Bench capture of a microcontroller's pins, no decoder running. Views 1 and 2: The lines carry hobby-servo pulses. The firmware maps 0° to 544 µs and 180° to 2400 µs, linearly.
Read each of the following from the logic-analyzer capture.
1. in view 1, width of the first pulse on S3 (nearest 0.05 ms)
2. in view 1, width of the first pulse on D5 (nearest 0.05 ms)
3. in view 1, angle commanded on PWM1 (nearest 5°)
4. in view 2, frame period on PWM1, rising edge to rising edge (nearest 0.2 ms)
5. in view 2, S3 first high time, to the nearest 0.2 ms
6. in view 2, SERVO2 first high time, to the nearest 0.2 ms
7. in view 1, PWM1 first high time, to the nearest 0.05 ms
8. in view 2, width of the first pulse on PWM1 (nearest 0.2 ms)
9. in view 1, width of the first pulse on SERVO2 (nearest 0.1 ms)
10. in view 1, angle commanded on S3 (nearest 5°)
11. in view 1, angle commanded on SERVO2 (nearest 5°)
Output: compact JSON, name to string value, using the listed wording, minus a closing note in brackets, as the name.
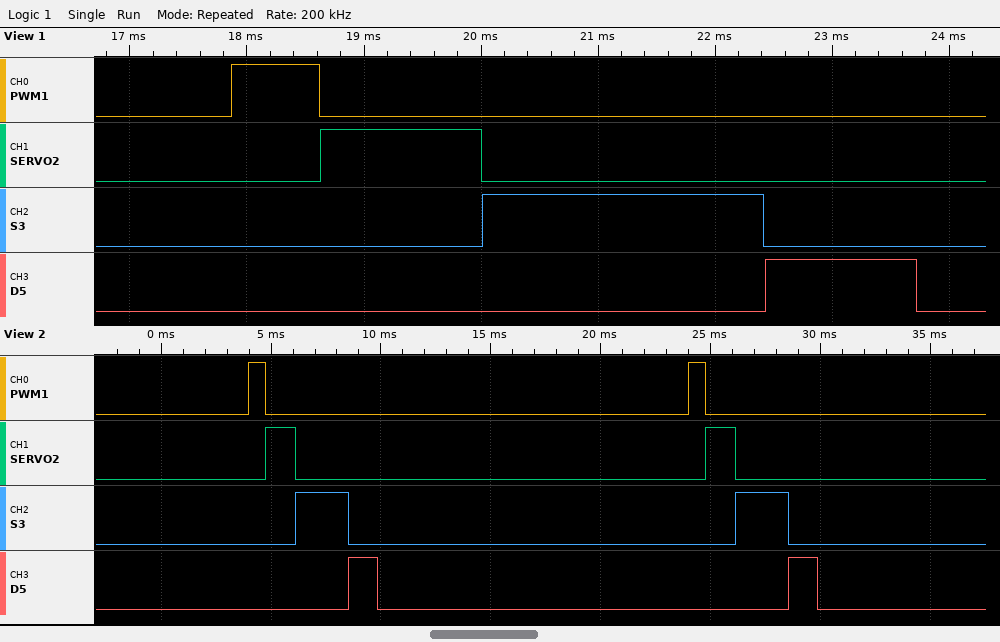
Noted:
{"in view 1, width of the first pulse on S3": "2.40 ms", "in view 1, width of the first pulse on D5": "1.30 ms", "in view 1, angle commanded on PWM1": "20°", "in view 2, frame period on PWM1, rising edge to rising edge": "20.0 ms", "in view 2, S3 first high time, to the nearest 0.2 ms": "2.4 ms", "in view 2, SERVO2 first high time, to the nearest 0.2 ms": "1.4 ms", "in view 1, PWM1 first high time, to the nearest 0.05 ms": "0.75 ms", "in view 2, width of the first pulse on PWM1": "0.8 ms", "in view 1, width of the first pulse on SERVO2": "1.4 ms", "in view 1, angle commanded on S3": "180°", "in view 1, angle commanded on SERVO2": "80°"}
